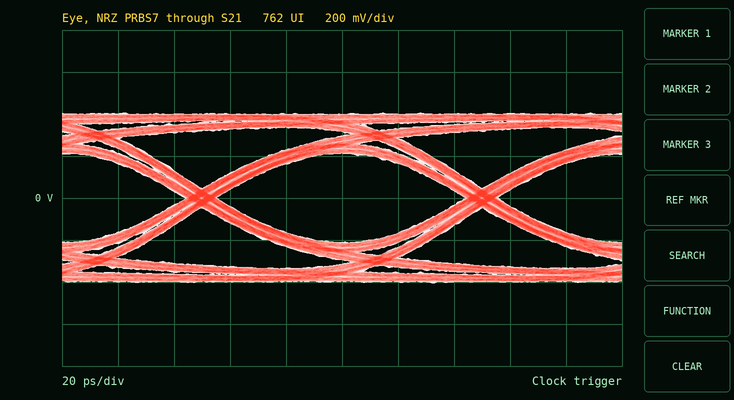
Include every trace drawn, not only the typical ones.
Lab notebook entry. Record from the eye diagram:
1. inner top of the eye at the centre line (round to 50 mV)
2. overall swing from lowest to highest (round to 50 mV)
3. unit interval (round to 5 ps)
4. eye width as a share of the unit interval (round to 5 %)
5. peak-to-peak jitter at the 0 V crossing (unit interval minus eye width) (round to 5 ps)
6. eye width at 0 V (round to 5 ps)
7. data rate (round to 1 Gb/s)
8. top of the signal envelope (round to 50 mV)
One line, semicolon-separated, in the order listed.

200 mV; 800 mV; 100 ps; 90 %; 10 ps; 90 ps; 10 Gb/s; 400 mV
